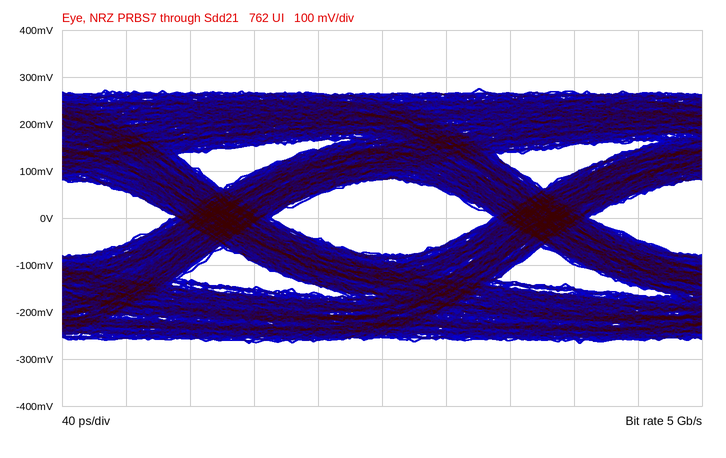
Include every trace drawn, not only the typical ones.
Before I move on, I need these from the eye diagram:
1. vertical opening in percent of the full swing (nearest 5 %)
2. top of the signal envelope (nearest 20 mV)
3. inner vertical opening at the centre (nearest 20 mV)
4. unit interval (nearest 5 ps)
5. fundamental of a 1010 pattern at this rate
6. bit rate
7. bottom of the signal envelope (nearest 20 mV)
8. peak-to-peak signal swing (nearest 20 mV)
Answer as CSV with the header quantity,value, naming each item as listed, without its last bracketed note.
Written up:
quantity,value
vertical opening in percent of the full swing,30 %
top of the signal envelope,280 mV
inner vertical opening at the centre,160 mV
unit interval,200 ps
fundamental of a 1010 pattern at this rate,2.5 GHz
bit rate,5 Gb/s
bottom of the signal envelope,-260 mV
peak-to-peak signal swing,540 mV
